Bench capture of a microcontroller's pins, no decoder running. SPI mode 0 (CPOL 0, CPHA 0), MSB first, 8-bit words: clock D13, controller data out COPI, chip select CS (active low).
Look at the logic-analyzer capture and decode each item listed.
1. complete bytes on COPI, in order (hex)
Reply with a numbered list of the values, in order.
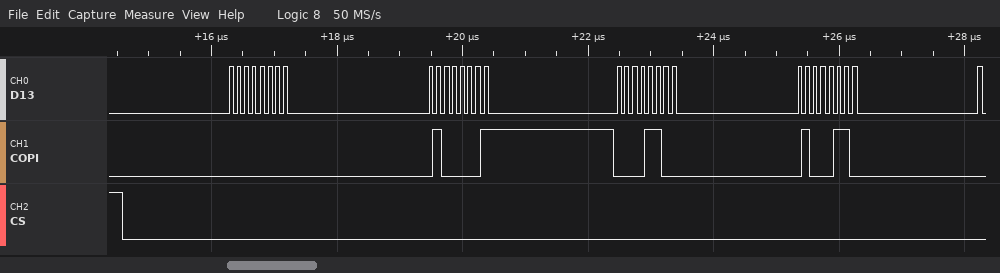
1. 00 41 0C 46
